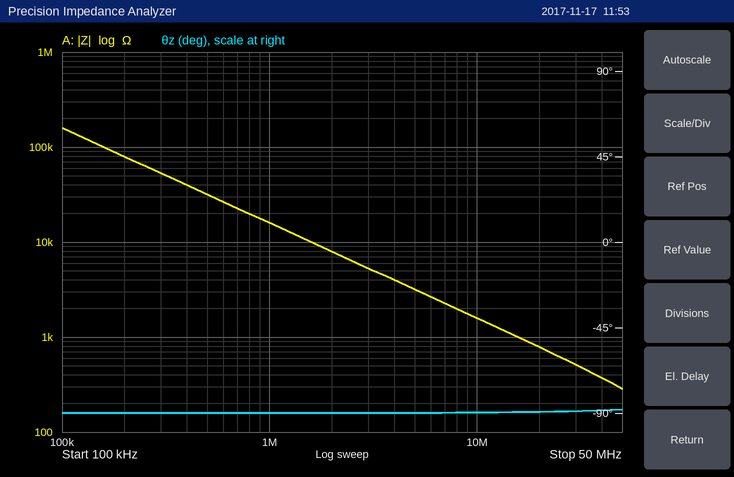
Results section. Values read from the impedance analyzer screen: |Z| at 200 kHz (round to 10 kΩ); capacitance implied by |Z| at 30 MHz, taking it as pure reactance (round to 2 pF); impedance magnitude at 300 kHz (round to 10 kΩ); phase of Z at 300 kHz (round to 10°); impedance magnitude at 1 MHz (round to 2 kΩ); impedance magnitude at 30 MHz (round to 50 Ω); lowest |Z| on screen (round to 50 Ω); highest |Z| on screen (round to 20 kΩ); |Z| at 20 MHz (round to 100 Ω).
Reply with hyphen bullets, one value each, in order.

- 80 kΩ
- 10 pF
- 50 kΩ
- -90°
- 16 kΩ
- 500 Ω
- 300 Ω
- 160 kΩ
- 800 Ω
